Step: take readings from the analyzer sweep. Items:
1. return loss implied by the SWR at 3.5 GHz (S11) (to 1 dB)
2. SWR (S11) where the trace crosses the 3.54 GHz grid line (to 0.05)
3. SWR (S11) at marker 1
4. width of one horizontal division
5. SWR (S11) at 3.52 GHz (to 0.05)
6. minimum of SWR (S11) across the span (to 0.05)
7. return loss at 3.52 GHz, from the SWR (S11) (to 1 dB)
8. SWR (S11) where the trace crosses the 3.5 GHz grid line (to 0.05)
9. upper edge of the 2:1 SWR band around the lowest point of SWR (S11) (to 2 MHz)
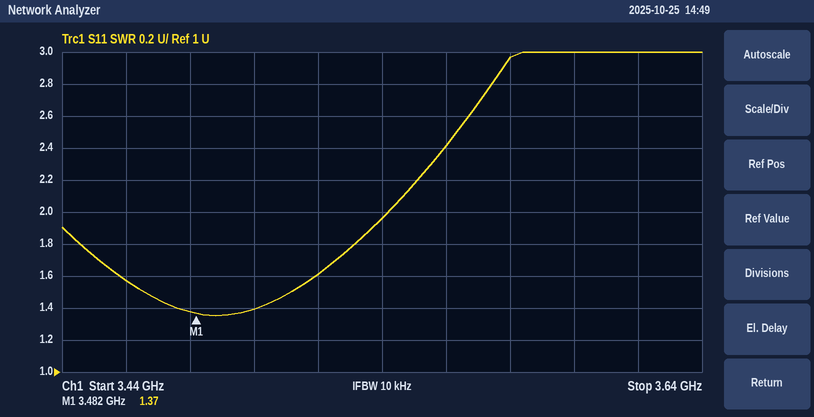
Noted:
16 dB
1.95
1.37
20 MHz
1.60
1.35
13 dB
1.40
3.542 GHz
